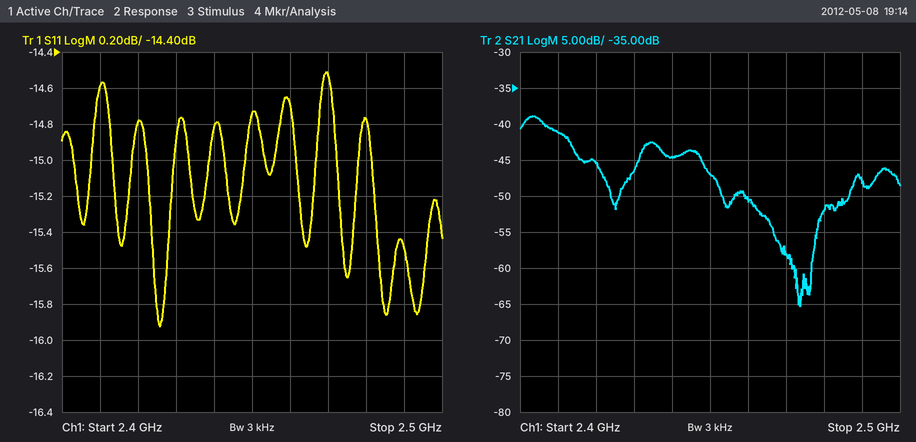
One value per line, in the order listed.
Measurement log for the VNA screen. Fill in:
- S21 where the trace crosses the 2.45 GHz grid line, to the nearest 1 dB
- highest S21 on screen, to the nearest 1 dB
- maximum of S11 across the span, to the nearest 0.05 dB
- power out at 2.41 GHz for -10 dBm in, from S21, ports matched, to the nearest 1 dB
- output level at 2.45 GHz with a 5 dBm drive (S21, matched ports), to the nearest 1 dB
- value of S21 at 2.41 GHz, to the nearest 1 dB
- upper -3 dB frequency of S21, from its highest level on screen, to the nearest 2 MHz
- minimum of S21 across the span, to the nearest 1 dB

-47 dB
-39 dB
-14.50 dB
-51 dBm
-42 dBm
-41 dB
2.412 GHz
-65 dB
